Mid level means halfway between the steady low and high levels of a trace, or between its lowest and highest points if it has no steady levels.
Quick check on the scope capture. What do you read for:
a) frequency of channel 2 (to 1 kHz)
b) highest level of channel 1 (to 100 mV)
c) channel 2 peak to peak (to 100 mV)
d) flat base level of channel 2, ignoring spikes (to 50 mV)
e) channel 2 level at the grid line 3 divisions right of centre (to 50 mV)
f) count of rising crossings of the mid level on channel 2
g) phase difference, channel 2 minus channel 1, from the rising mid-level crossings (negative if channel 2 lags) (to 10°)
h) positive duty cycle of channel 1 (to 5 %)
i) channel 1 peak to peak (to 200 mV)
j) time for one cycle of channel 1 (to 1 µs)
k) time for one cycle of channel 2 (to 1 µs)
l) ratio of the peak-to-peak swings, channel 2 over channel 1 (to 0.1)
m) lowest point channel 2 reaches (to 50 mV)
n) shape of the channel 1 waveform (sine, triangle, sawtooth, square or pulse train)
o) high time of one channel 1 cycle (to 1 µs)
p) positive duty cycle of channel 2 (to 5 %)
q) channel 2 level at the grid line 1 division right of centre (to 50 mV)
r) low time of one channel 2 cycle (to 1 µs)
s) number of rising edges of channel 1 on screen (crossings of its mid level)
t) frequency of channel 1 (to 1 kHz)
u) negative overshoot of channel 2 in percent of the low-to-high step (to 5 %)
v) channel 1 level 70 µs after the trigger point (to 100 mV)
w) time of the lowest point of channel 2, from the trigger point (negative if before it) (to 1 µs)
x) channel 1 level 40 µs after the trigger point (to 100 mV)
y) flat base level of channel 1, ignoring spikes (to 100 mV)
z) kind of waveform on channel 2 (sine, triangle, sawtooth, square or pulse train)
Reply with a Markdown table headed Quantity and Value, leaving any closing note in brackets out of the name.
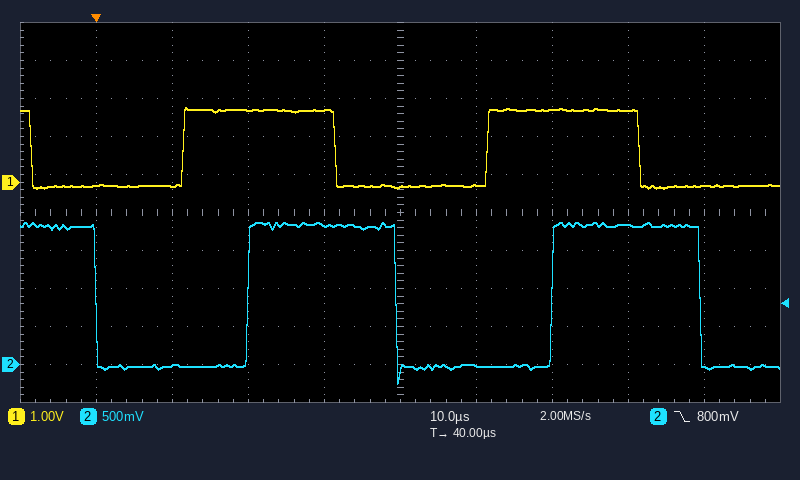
| Quantity | Value |
|---|---|
| frequency of channel 2 | 25 kHz |
| highest level of channel 1 | 2.0 V |
| channel 2 peak to peak | 2.10 V |
| flat base level of channel 2, ignoring spikes | -50 mV |
| channel 2 level at the grid line 3 divisions right of centre | 1.85 V |
| count of rising crossings of the mid level on channel 2 | 2 |
| phase difference, channel 2 minus channel 1, from the rising mid-level crossings (negative if channel 2 lags) | -80° |
| positive duty cycle of channel 1 | 50 % |
| channel 1 peak to peak | 2.2 V |
| time for one cycle of channel 1 | 40 µs |
| time for one cycle of channel 2 | 40 µs |
| ratio of the peak-to-peak swings, channel 2 over channel 1 | 1.0 |
| lowest point channel 2 reaches | -250 mV |
| shape of the channel 1 waveform | square |
| high time of one channel 1 cycle | 20 µs |
| positive duty cycle of channel 2 | 50 % |
| channel 2 level at the grid line 1 division right of centre | 0 mV |
| low time of one channel 2 cycle | 20 µs |
| number of rising edges of channel 1 on screen | 2 |
| frequency of channel 1 | 25 kHz |
| negative overshoot of channel 2 in percent of the low-to-high step | 10 % |
| channel 1 level 70 µs after the trigger point | 1.9 V |
| time of the lowest point of channel 2, from the trigger point (negative if before it) | +40 µs |
| channel 1 level 40 µs after the trigger point | -100 mV |
| flat base level of channel 1, ignoring spikes | -100 mV |
| kind of waveform on channel 2 | square |
